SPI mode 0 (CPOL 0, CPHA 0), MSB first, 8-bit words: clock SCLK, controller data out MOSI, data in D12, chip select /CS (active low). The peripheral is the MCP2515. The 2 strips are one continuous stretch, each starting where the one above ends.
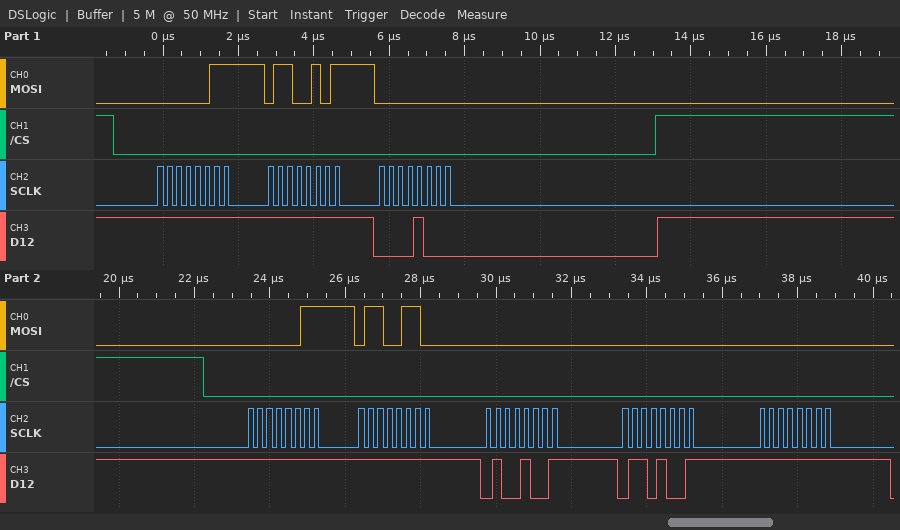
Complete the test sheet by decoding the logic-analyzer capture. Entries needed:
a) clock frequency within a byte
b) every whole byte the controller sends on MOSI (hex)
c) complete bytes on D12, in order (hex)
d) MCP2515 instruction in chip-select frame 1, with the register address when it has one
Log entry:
4 MHz
03 65 00 03 66 00 00 00
FF FF 08 FF FF 49 69 FF
READ 0x65
